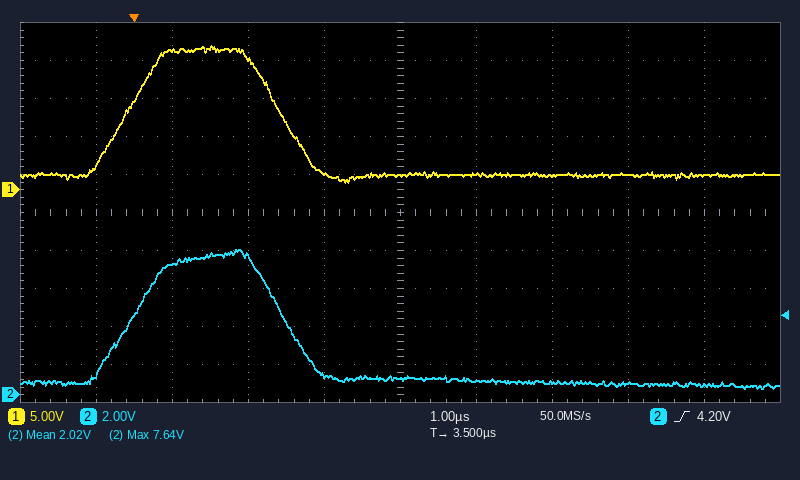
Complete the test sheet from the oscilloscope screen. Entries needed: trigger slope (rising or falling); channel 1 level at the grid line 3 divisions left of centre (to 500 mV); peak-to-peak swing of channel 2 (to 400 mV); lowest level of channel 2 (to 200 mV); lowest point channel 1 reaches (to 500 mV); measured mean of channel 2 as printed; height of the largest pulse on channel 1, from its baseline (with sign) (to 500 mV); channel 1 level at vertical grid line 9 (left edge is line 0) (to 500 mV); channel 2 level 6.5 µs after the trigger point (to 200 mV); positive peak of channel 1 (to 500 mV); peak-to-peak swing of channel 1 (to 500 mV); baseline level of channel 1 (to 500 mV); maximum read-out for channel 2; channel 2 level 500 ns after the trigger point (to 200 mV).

rising
18.5 V
7.2 V
400 mV
1.0 V
2.02 V
+17.0 V
2.0 V
600 mV
19.0 V
18.0 V
2.0 V
7.64 V
6.8 V
